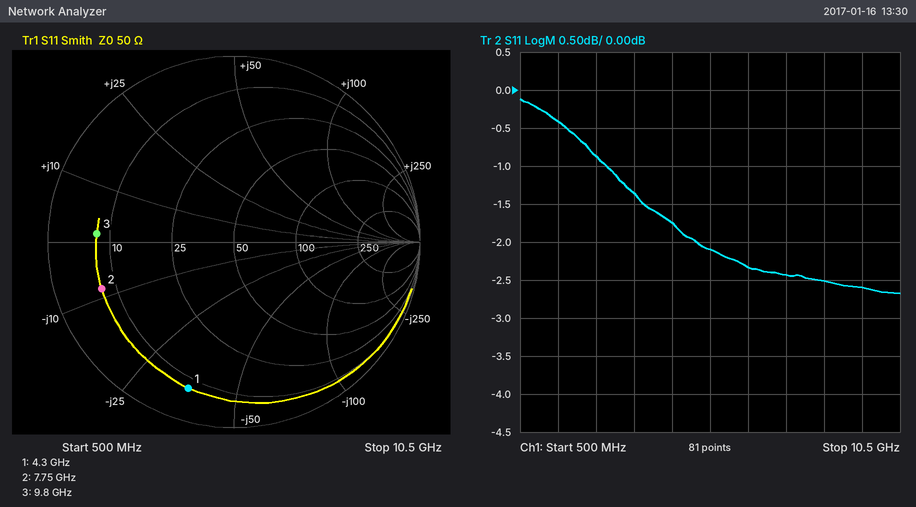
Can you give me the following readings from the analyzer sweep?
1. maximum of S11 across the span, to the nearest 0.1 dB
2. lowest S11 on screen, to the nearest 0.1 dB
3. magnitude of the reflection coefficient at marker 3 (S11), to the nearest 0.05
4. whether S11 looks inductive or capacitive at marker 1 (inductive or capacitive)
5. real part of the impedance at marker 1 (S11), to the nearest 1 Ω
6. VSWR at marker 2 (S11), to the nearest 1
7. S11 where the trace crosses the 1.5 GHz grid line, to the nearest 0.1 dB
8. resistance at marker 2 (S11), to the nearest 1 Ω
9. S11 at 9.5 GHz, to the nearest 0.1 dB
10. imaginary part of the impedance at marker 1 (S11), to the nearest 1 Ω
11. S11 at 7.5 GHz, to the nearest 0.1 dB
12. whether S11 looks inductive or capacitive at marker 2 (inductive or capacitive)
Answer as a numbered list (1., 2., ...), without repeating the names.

1. -0.1 dB
2. -2.7 dB
3. 0.75
4. capacitive
5. 7 Ω
6. 7
7. -0.4 dB
8. 7 Ω
9. -2.6 dB
10. -36 Ω
11. -2.4 dB
12. capacitive
